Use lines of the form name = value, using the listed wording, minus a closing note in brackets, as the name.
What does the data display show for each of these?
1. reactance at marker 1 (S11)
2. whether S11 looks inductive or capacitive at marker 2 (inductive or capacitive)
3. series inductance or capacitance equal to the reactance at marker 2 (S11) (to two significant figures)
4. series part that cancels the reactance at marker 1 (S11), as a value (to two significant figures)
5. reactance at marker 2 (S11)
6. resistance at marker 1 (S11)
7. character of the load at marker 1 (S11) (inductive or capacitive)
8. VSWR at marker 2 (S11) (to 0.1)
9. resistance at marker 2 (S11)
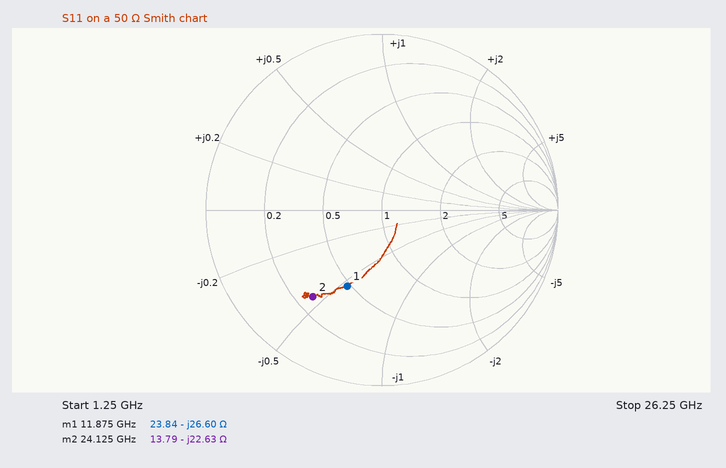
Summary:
reactance at marker 1 = -26.60 Ω
whether S11 looks inductive or capacitive at marker 2 = capacitive
series inductance or capacitance equal to the reactance at marker 2 (S11) = 290 fF
series part that cancels the reactance at marker 1 (S11), as a value = 360 pH
reactance at marker 2 = -22.63 Ω
resistance at marker 1 = 23.84 Ω
character of the load at marker 1 (S11) = capacitive
VSWR at marker 2 (S11) = 4.4
resistance at marker 2 = 13.79 Ω
